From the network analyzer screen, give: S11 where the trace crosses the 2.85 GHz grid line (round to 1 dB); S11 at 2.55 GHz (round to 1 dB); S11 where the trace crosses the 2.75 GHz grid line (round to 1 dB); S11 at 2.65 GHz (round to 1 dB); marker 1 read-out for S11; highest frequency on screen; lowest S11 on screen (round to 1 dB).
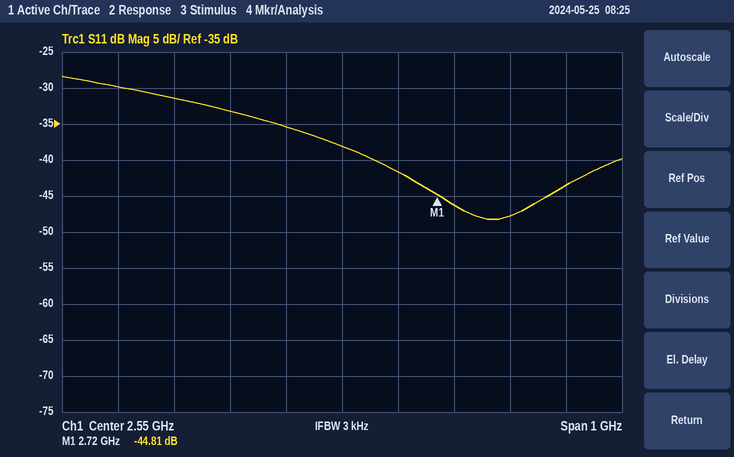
-48 dB
-38 dB
-46 dB
-42 dB
-44.81 dB
3.05 GHz
-48 dB
